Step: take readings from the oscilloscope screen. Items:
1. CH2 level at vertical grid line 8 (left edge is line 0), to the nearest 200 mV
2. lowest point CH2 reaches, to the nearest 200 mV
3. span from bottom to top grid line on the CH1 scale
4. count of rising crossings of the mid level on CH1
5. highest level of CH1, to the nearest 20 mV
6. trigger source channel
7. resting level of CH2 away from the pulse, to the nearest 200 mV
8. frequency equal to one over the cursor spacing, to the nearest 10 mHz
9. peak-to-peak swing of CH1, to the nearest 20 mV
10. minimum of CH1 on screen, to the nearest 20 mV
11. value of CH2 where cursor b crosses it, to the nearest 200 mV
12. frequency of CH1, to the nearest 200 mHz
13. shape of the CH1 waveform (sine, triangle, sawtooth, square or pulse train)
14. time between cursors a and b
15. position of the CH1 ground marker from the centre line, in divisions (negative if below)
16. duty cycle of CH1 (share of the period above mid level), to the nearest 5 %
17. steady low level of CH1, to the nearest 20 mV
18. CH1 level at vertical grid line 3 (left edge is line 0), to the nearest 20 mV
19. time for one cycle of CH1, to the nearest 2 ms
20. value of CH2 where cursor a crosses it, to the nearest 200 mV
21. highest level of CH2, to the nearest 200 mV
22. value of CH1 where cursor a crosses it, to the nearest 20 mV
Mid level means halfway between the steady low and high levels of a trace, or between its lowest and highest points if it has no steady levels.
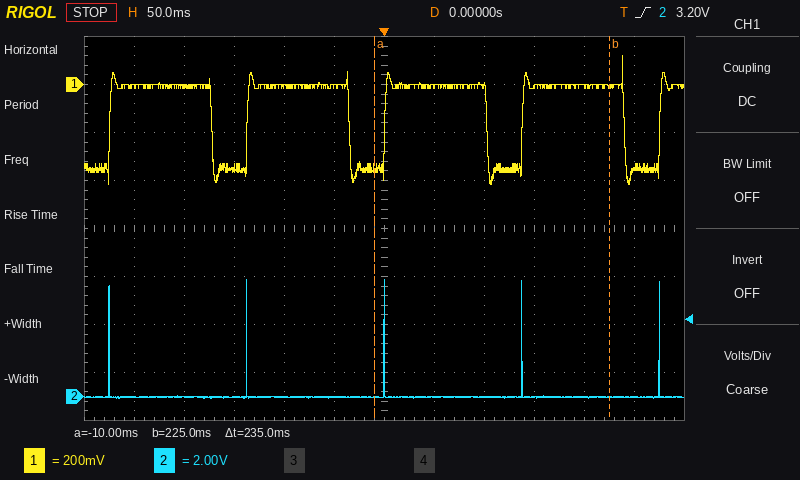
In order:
0.0 V
0.0 V
1.6 V
5
120 mV
CH2
0.0 V
4.26 Hz
540 mV
-420 mV
0.0 V
7.2 Hz
pulse train
235 ms
+3.0 div
75 %
-360 mV
-340 mV
138 ms
0.0 V
4.8 V
-340 mV
